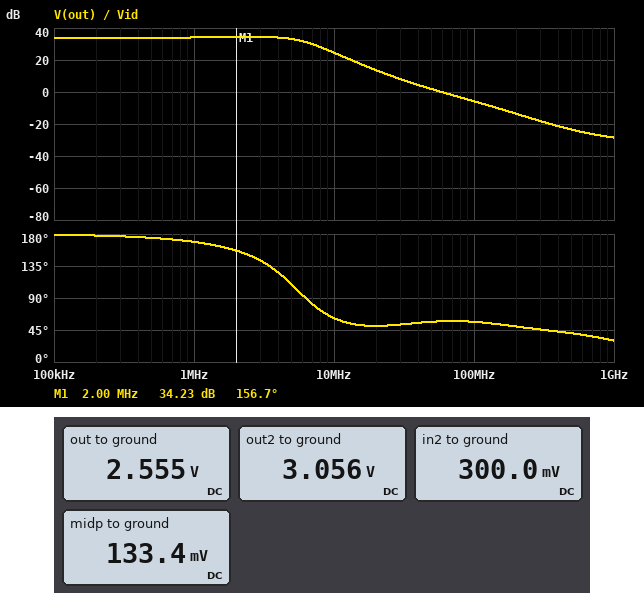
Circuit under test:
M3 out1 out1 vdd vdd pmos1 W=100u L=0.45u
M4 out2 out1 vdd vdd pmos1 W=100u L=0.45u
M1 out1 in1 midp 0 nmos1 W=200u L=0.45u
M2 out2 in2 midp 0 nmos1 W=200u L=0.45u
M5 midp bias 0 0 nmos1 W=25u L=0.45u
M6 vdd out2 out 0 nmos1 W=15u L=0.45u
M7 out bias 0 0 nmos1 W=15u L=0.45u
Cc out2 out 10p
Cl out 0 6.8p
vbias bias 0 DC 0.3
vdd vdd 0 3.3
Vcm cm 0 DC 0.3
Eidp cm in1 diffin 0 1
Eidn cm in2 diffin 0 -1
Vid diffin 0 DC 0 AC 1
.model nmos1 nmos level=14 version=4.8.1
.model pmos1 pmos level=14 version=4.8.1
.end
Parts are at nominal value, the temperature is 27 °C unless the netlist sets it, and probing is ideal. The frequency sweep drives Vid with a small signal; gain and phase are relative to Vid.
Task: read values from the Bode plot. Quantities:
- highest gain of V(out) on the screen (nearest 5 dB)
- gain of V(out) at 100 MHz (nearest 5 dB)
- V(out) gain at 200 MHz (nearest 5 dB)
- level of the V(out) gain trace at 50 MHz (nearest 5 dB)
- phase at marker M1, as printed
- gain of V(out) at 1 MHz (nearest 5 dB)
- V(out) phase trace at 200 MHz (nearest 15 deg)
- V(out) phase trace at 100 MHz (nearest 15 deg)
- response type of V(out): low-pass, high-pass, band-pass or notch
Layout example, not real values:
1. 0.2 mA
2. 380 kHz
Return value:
1. 35 dB
2. -5 dB
3. -15 dB
4. 0 dB
5. 156.7 deg
6. 35 dB
7. 45 deg
8. 60 deg
9. low-pass
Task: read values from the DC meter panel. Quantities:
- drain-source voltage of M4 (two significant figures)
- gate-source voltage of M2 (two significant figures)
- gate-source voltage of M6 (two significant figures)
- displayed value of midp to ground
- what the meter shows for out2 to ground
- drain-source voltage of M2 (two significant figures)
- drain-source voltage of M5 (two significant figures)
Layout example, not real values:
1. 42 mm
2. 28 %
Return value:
1. -240 mV
2. 170 mV
3. 500 mV
4. 133.4 mV
5. 3.056 V
6. 2.9 V
7. 130 mV
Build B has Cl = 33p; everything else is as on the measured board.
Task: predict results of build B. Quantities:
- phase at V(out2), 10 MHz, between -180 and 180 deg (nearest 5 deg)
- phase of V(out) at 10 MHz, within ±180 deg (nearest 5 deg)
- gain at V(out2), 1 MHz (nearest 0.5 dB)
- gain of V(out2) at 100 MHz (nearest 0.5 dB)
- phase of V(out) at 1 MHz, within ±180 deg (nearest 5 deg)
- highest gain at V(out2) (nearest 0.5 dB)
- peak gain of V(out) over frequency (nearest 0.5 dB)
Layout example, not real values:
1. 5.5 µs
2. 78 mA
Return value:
1. 65 deg
2. 30 deg
3. 35.5 dB
4. -6.5 dB
5. 160 deg
6. 37.5 dB
7. 36.5 dB
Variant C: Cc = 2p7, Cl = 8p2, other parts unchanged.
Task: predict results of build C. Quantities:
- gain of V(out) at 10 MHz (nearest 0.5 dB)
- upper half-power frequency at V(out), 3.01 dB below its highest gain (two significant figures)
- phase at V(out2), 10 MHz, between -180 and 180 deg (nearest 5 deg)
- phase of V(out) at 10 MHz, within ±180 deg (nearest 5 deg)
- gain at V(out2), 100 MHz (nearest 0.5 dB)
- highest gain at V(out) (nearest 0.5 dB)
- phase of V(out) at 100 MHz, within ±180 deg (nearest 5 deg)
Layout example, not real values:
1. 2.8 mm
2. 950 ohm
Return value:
1. 31.0 dB
2. 9.8 MHz
3. 100 deg
4. 85 deg
5. 3.5 dB
6. 34.0 dB
7. 30 deg
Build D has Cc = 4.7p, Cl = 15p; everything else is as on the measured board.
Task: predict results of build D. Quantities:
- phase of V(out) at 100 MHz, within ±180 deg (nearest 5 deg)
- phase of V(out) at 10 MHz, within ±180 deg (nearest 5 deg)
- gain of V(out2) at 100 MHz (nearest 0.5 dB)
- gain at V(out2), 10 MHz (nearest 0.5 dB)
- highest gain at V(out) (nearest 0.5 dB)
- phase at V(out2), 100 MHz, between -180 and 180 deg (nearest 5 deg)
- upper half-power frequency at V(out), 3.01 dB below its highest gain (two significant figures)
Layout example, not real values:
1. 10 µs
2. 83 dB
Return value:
1. 40 deg
2. 45 deg
3. -0.5 dB
4. 26.5 dB
5. 35.0 dB
6. 65 deg
7. 6.3 MHz
